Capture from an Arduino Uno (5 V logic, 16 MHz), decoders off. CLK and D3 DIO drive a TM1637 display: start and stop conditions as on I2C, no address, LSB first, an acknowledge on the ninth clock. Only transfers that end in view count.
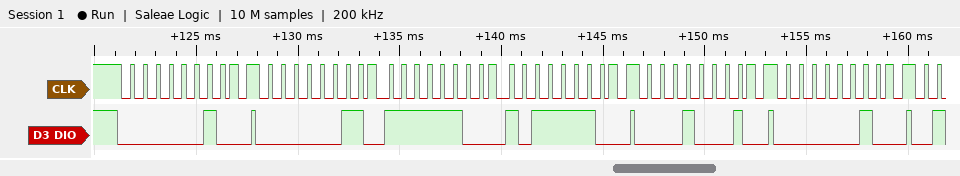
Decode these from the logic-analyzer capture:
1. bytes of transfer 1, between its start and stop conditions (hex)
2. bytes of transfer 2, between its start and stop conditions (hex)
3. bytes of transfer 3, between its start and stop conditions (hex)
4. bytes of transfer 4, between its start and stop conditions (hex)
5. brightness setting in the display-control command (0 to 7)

40
C0 3F 7D
88
40
0
